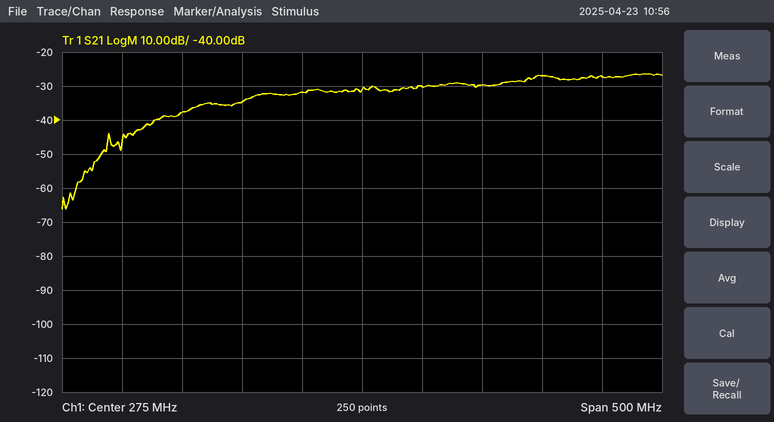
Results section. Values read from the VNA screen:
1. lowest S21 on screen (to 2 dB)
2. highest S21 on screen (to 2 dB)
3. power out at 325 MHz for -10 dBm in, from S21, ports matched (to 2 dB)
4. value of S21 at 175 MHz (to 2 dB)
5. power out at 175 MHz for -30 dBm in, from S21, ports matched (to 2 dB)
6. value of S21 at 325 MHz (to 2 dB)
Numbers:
-66 dB
-26 dB
-40 dBm
-34 dB
-64 dBm
-30 dB
